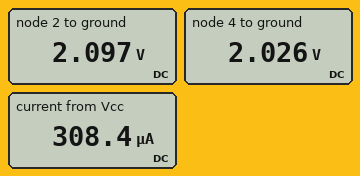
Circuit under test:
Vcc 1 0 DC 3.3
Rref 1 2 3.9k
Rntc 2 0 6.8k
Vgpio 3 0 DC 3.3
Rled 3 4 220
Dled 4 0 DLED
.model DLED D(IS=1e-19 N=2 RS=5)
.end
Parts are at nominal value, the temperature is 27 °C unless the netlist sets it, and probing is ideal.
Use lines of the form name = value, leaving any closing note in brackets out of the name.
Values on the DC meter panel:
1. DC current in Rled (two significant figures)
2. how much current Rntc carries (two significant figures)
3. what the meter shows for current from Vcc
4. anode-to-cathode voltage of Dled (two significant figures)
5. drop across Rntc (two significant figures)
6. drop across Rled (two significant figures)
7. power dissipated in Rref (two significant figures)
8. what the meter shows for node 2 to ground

DC current in Rled = 5.8 mA
how much current Rntc carries = 310 µA
what the meter shows for current from Vcc = 308.4 µA
anode-to-cathode voltage of Dled = 2.0 V
drop across Rntc = 2.1 V
drop across Rled = 1.3 V
power dissipated in Rref = 370 µW
what the meter shows for node 2 to ground = 2.097 V
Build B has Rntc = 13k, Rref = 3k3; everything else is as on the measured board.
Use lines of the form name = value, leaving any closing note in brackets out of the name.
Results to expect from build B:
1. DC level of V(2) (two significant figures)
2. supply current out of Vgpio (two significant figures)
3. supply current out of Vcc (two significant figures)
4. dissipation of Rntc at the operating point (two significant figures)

DC level of V(2) = 2.6 V
supply current out of Vgpio = 5.8 mA
supply current out of Vcc = 200 µA
dissipation of Rntc at the operating point = 530 µW
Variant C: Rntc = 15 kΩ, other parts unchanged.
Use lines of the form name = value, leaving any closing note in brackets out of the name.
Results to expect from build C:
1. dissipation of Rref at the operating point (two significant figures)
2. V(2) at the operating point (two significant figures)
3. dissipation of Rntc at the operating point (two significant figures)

dissipation of Rref at the operating point = 120 µW
V(2) at the operating point = 2.6 V
dissipation of Rntc at the operating point = 460 µW
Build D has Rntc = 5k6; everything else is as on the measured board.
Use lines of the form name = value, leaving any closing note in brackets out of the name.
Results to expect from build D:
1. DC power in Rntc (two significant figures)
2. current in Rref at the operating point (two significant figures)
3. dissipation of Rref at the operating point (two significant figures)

DC power in Rntc = 680 µW
current in Rref at the operating point = 350 µA
dissipation of Rref at the operating point = 470 µW
